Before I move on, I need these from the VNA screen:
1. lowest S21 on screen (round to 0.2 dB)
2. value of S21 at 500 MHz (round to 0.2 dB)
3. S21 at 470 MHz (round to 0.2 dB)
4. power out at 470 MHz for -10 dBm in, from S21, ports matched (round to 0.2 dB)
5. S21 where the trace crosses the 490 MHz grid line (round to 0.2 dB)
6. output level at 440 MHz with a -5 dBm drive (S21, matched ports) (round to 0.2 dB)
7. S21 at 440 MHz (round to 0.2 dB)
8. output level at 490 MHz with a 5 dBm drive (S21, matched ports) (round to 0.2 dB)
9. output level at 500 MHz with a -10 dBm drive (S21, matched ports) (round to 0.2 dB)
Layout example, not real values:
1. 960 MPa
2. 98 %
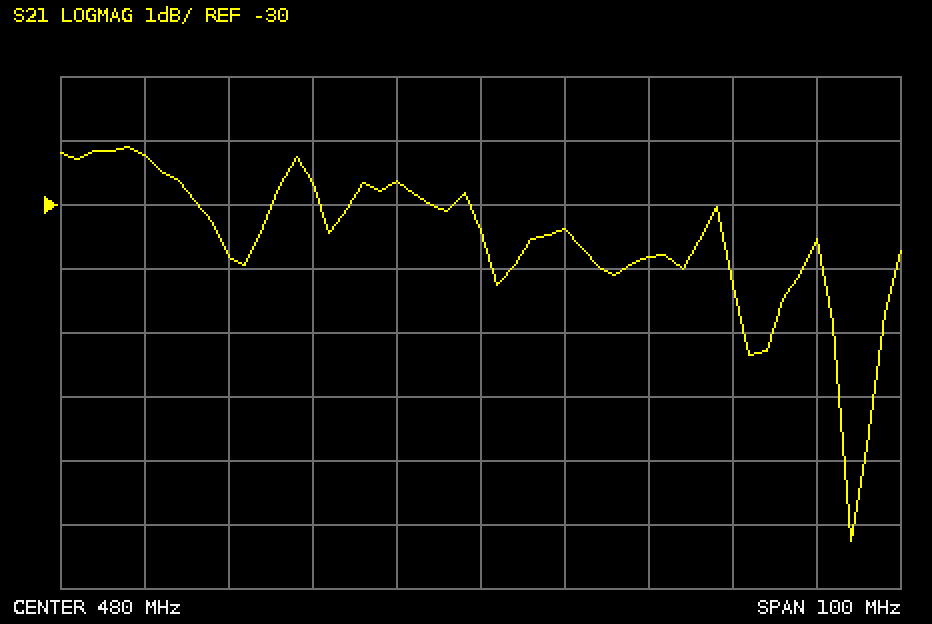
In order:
1. -35.2 dB
2. -30.8 dB
3. -29.6 dB
4. -39.6 dBm
5. -30.4 dB
6. -34.2 dBm
7. -29.2 dB
8. -25.4 dBm
9. -40.8 dBm
